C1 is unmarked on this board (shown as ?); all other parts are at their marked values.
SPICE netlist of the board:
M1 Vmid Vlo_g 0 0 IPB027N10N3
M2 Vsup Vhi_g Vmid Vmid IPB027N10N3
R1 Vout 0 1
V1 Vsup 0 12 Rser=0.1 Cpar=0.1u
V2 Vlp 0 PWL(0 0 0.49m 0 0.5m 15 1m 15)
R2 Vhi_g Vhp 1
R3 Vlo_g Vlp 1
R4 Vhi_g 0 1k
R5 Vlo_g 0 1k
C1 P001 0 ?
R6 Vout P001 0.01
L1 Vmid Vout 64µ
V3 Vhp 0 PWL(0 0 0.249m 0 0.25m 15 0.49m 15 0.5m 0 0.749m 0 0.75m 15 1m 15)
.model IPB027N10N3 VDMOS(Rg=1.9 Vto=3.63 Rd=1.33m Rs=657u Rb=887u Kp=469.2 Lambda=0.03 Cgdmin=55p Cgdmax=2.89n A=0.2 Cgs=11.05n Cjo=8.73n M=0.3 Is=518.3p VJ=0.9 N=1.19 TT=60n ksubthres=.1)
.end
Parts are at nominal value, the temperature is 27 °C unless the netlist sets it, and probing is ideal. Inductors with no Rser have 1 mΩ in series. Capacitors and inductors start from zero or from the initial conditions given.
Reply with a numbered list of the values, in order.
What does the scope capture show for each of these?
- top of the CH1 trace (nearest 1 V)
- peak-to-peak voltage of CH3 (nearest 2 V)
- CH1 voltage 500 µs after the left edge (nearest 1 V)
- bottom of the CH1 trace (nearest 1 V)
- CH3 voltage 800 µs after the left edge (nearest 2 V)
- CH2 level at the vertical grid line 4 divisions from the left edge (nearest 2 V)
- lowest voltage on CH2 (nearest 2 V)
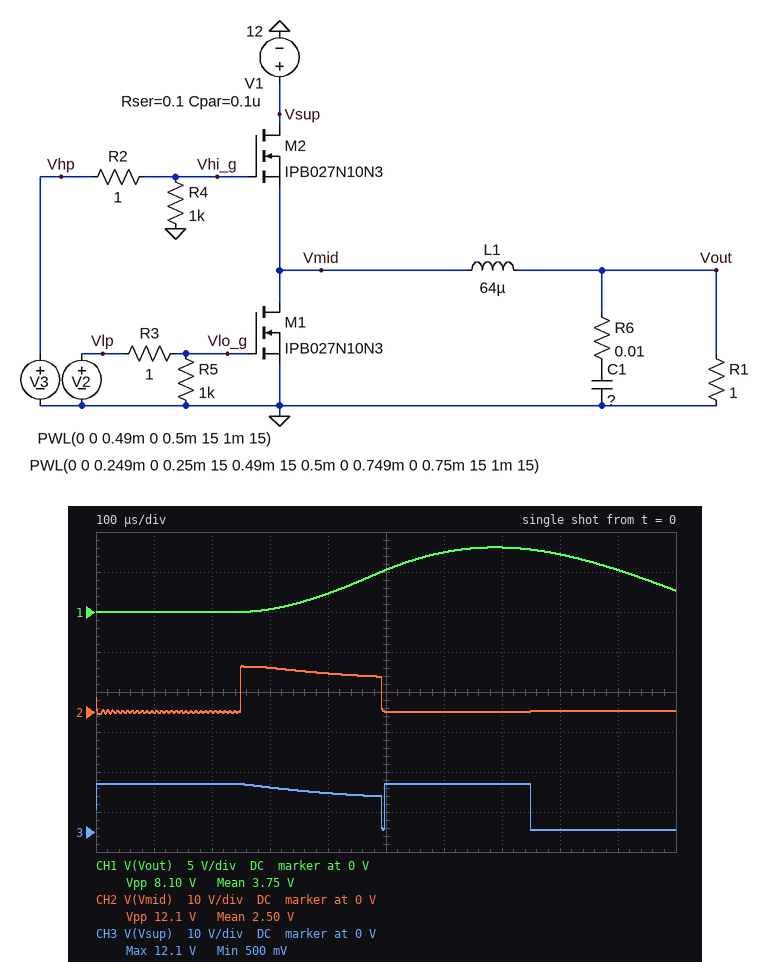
1. 8 V
2. 12 V
3. 5 V
4. 0 V
5. 0 V
6. 10 V
7. 0 V
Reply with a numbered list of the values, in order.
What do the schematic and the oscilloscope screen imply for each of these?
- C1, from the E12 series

1. 820 µF
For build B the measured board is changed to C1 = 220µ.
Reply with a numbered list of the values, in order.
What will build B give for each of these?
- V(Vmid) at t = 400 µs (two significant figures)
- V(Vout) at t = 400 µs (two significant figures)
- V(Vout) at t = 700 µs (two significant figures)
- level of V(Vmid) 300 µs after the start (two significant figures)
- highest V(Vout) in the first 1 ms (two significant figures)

1. 10 V
2. 6.3 V
3. 4.5 V
4. 11 V
5. 12 V
